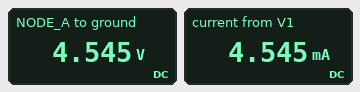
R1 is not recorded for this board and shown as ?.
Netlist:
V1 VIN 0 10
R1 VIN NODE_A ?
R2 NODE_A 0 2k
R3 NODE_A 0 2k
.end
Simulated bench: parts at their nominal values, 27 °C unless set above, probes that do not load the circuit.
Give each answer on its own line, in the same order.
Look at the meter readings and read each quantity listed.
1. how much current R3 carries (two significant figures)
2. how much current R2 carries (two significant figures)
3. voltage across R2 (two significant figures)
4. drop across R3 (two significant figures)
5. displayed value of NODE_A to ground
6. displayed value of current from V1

2.3 mA
2.3 mA
4.5 V
4.5 V
4.545 V
4.545 mA
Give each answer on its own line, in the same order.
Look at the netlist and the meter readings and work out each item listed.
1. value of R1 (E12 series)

1.2 kΩ
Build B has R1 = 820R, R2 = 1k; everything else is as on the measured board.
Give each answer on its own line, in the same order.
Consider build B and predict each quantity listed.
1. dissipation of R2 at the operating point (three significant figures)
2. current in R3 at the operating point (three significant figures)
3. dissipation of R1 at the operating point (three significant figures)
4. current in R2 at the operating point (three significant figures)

20.1 mW
2.24 mA
37.1 mW
4.48 mA
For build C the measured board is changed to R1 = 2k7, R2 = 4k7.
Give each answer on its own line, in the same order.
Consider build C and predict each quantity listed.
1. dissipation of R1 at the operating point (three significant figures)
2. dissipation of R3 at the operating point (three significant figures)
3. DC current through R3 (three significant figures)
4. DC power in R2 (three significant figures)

16.0 mW
5.85 mW
1.71 mA
2.49 mW
